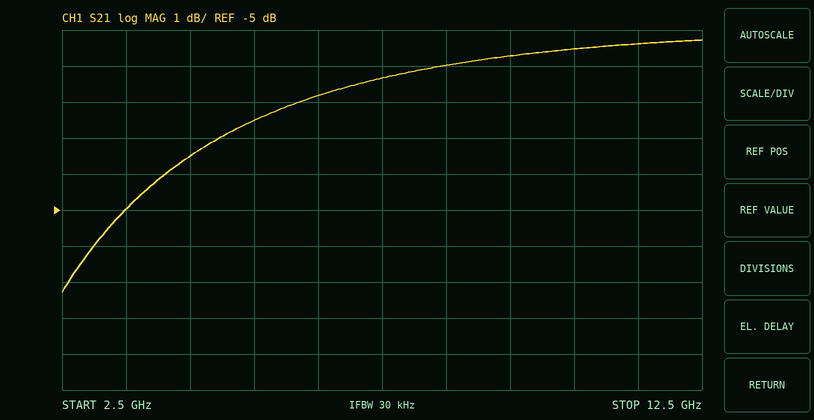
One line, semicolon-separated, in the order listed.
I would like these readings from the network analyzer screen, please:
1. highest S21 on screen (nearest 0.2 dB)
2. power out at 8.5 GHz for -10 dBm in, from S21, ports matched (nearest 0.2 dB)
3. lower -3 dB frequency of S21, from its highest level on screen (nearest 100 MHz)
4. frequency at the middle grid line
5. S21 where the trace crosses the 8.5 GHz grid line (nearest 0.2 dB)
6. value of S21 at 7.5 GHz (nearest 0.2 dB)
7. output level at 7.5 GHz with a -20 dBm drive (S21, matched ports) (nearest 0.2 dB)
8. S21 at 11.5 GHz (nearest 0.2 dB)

-0.2 dB; -11.0 dBm; 4.7 GHz; 7.5 GHz; -1.0 dB; -1.4 dB; -21.4 dBm; -0.4 dB
